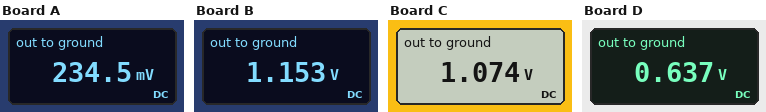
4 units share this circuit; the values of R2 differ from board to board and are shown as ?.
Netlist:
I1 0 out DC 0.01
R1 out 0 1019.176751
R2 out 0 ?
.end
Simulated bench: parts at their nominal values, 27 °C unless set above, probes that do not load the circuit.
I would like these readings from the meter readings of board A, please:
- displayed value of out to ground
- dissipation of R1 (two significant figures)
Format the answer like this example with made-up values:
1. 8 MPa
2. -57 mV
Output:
1. 234.5 mV
2. 54 µW
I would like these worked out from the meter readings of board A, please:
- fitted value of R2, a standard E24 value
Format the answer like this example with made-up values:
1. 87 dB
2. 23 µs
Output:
1. 24 Ω
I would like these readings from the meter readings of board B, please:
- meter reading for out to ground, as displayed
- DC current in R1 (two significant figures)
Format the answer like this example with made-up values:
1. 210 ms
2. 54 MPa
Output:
1. 1.153 V
2. 1.1 mA
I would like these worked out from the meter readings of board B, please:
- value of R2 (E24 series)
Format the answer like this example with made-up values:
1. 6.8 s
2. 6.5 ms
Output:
1. 130 Ω
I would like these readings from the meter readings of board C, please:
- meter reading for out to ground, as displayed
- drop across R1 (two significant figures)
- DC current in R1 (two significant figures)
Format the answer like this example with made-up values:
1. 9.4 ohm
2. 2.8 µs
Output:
1. 1.074 V
2. 1.1 V
3. 1.1 mA
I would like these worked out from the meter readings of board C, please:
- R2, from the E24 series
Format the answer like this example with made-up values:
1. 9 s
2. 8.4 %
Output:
1. 120 Ω
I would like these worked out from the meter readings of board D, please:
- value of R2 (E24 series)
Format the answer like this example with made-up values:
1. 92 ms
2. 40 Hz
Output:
1. 68 Ω
